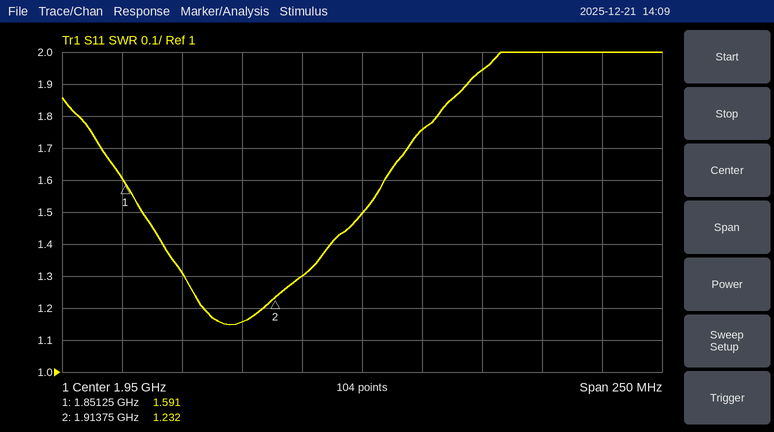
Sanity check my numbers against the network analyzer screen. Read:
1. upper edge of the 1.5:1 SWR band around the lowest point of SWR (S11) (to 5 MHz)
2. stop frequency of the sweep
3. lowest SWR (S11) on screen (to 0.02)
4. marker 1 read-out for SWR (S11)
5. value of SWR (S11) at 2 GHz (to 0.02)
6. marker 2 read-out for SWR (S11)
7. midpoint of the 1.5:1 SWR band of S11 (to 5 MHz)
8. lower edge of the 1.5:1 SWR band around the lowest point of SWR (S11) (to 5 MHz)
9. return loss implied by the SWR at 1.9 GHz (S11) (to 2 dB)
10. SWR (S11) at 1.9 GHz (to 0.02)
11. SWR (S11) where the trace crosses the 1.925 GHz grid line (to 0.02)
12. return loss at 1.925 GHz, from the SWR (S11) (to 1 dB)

1.950 GHz
2.075 GHz
1.14
1.591
1.94
1.232
1.905 GHz
1.860 GHz
22 dB
1.16
1.30
18 dB
